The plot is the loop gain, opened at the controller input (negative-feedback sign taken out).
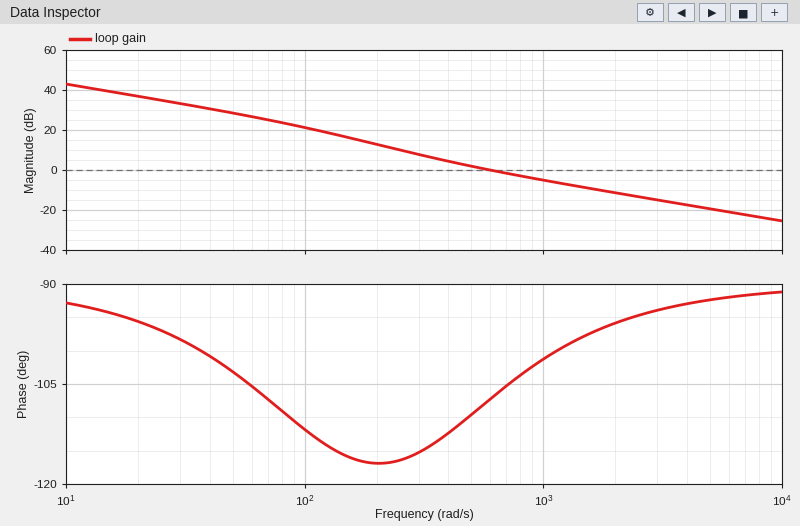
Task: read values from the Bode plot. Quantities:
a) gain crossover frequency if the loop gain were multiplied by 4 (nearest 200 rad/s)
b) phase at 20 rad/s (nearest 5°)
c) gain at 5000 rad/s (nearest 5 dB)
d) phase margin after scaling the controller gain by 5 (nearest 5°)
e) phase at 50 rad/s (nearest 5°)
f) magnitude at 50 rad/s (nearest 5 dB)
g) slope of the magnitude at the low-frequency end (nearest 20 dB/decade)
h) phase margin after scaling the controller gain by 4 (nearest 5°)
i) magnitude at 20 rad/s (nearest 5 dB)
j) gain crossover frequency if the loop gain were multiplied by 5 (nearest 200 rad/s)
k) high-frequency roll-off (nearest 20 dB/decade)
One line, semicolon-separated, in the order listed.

2200 rad/s; -95°; -20 dB; 85°; -105°; 30 dB; -20 dB/decade; 85°; 35 dB; 2600 rad/s; -20 dB/decade
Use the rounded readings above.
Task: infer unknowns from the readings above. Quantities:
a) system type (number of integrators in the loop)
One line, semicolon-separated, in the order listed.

1
